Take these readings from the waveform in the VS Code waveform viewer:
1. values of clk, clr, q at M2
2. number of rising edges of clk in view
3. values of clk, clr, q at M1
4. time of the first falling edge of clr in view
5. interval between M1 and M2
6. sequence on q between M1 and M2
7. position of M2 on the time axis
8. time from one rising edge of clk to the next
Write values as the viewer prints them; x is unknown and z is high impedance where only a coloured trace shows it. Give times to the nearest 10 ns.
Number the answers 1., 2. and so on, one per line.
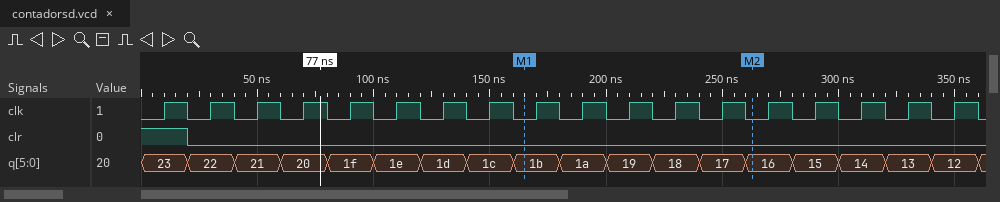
1. clk=0, clr=0, q=16
2. 18
3. clk=0, clr=0, q=1b
4. 20 ns
5. 100 ns
6. 1b, 1a, 19, 18, 17, 16
7. 260 ns
8. 20 ns
